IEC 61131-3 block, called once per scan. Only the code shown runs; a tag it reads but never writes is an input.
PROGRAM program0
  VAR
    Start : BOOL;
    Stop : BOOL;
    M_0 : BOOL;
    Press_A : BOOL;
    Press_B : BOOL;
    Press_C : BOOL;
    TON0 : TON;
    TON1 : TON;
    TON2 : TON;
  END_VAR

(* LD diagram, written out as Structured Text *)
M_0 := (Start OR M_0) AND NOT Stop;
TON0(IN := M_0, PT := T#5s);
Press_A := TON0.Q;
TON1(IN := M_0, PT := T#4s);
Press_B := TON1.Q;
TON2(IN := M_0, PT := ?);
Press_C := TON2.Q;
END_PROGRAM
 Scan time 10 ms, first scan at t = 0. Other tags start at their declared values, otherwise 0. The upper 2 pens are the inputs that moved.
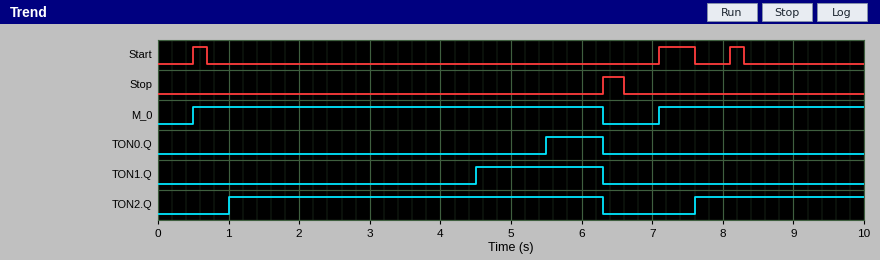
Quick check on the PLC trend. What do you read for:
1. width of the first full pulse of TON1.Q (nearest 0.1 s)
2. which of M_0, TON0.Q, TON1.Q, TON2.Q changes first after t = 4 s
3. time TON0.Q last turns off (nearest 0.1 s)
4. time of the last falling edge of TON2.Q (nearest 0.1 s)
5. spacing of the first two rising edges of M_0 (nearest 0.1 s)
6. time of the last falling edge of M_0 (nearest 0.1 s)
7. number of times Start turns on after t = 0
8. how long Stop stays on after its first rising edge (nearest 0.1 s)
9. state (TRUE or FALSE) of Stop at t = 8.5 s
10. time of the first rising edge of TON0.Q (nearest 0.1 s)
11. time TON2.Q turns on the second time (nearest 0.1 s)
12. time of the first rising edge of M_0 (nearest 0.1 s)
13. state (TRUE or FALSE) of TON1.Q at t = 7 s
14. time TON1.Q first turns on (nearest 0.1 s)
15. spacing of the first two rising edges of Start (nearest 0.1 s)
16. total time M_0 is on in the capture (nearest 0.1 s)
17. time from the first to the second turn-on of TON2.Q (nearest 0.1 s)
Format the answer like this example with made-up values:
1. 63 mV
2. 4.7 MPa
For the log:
1. 1.8 s
2. TON1.Q
3. 6.3 s
4. 6.3 s
5. 6.6 s
6. 6.3 s
7. 3
8. 0.3 s
9. FALSE
10. 5.5 s
11. 7.6 s
12. 0.5 s
13. FALSE
14. 4.5 s
15. 6.6 s
16. 8.7 s
17. 6.6 s
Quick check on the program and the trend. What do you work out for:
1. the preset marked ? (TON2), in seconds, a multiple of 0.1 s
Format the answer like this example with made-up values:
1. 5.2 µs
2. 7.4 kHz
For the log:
1. 0.5 s
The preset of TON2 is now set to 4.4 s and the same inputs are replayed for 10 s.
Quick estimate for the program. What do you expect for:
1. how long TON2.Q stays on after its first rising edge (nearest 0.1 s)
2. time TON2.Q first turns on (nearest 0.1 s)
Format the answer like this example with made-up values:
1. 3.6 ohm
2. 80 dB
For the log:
1. 1.4 s
2. 4.9 s
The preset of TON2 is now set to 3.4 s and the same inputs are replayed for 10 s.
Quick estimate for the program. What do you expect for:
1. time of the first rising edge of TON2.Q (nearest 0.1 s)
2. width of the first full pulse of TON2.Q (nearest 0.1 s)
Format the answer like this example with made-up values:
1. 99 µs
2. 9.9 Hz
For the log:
1. 3.9 s
2. 2.4 s
